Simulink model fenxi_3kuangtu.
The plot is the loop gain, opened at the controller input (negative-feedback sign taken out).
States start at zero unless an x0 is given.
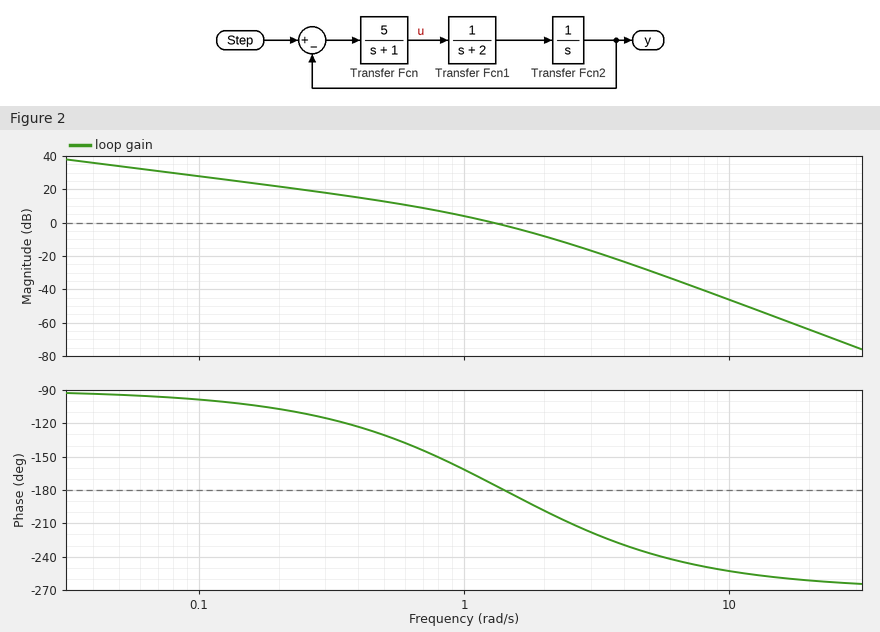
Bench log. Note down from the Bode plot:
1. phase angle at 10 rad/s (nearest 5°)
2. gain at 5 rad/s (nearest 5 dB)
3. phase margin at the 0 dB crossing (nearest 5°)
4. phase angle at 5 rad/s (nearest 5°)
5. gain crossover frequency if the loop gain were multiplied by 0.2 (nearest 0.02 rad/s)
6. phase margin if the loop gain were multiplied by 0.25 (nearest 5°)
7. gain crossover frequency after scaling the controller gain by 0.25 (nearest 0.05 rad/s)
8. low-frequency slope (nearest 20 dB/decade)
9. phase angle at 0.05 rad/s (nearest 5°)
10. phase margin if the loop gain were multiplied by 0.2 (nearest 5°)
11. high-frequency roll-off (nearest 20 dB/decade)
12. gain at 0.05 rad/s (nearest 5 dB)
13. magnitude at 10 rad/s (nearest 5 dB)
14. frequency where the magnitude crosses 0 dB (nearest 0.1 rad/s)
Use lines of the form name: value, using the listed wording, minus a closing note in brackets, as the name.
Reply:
phase angle at 10 rad/s: -255°
gain at 5 rad/s: -30 dB
phase margin at the 0 dB crossing: 5°
phase angle at 5 rad/s: -235°
gain crossover frequency if the loop gain were multiplied by 0.2: 0.44 rad/s
phase margin if the loop gain were multiplied by 0.25: 45°
gain crossover frequency after scaling the controller gain by 0.25: 0.55 rad/s
low-frequency slope: -20 dB/decade
phase angle at 0.05 rad/s: -95°
phase margin if the loop gain were multiplied by 0.2: 55°
high-frequency roll-off: -60 dB/decade
gain at 0.05 rad/s: 35 dB
magnitude at 10 rad/s: -45 dB
frequency where the magnitude crosses 0 dB: 1.3 rad/s
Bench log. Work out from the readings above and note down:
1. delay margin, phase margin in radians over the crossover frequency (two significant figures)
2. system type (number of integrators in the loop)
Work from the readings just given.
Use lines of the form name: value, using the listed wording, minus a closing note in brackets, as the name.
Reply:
delay margin, phase margin in radians over the crossover frequency: 0.067 s
system type: 1
